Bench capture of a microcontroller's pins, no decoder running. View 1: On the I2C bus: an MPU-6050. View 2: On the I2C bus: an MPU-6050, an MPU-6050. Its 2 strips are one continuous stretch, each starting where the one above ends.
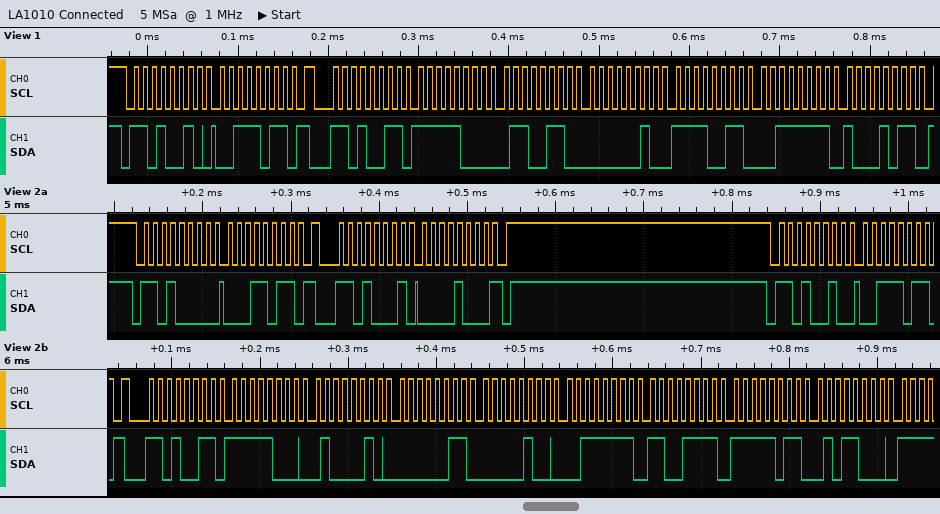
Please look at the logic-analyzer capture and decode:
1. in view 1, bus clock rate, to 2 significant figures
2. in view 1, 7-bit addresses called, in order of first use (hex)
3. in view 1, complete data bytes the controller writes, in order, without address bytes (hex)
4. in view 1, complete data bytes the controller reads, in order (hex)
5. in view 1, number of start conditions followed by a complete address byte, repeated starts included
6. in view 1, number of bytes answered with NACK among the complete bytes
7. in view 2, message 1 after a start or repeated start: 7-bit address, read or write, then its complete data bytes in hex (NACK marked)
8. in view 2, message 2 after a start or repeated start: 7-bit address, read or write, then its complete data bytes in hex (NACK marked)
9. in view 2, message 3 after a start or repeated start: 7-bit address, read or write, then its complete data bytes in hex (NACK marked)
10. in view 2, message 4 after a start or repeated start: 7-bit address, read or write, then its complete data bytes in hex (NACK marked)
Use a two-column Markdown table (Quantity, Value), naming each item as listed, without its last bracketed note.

| Quantity | Value |
|---|---|
| in view 1, bus clock rate, to 2 significant figures | 100 kHz |
| in view 1, 7-bit addresses called, in order of first use | 0x69 |
| in view 1, complete data bytes the controller writes, in order, without address bytes | 3B |
| in view 1, complete data bytes the controller reads, in order | F8 66 02 F3 3F 8B |
| in view 1, number of start conditions followed by a complete address byte, repeated starts included | 2 |
| in view 1, number of bytes answered with NACK among the complete bytes | 0 |
| in view 2, message 1 after a start or repeated start: 7-bit address, read or write, then its complete data bytes in hex | 0x68 write: 1B |
| in view 2, message 2 after a start or repeated start: 7-bit address, read or write, then its complete data bytes in hex | 0x68 read: 08 NACK |
| in view 2, message 3 after a start or repeated start: 7-bit address, read or write, then its complete data bytes in hex | 0x69 write: 3B |
| in view 2, message 4 after a start or repeated start: 7-bit address, read or write, then its complete data bytes in hex | 0x69 read: F8 42 03 04 3F CF FB 58 |
